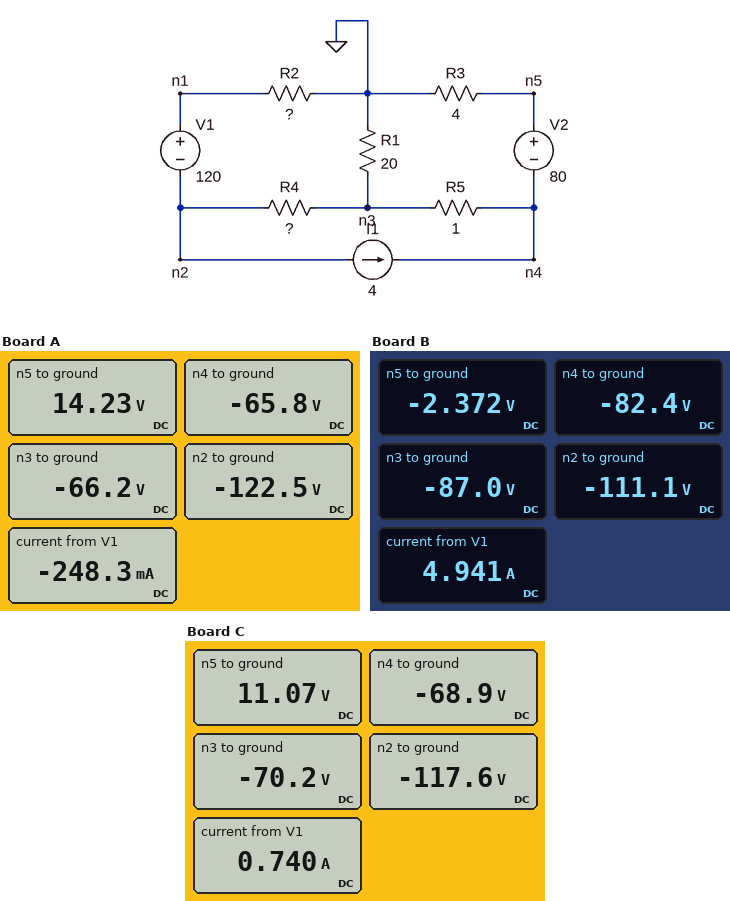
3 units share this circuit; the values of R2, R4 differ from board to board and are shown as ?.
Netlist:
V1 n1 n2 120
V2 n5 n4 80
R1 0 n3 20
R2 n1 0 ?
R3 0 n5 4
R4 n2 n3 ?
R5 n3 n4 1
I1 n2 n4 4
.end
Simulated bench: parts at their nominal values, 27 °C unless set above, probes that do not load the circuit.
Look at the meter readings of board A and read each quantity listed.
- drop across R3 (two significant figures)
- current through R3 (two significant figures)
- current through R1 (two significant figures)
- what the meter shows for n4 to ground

14 V
3.6 A
3.3 A
-65.8 V
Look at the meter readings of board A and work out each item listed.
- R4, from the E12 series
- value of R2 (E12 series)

15 Ω
10 Ω
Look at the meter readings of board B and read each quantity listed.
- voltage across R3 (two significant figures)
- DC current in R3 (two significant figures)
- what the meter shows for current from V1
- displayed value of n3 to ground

2.4 V
590 mA
4.941 A
-87.0 V
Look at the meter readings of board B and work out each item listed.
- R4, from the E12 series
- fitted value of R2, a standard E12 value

2.7 Ω
1.8 Ω
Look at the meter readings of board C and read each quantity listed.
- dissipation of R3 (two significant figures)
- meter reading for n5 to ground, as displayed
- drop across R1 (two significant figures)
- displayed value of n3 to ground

31 W
11.07 V
70 V
-70.2 V
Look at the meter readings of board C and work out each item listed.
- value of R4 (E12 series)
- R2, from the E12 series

10 Ω
3.3 Ω
